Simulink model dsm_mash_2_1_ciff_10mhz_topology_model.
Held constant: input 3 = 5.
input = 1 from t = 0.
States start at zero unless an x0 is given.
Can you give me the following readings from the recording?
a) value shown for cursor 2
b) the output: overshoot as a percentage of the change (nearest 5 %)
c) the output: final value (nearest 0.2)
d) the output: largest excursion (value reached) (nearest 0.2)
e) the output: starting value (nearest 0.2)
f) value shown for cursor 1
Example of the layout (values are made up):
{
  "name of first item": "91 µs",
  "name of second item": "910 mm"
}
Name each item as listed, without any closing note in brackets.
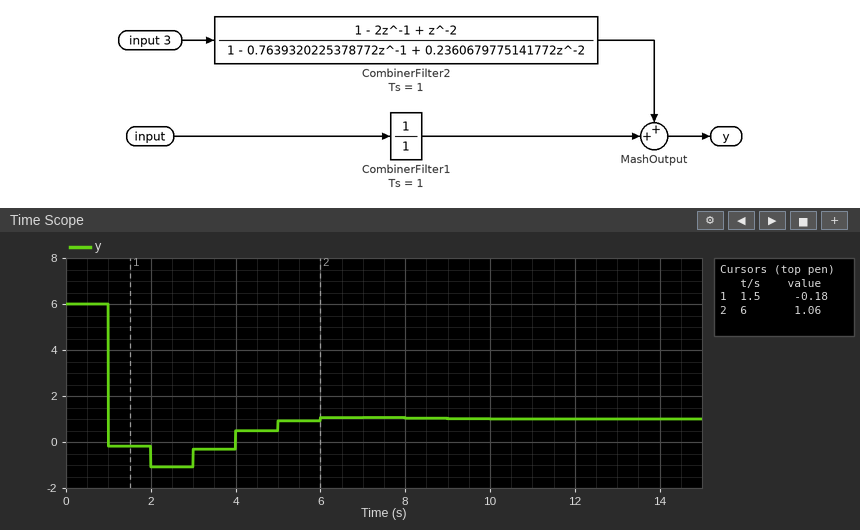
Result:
{
  "value shown for cursor 2": "1.06",
  "the output: overshoot as a percentage of the change": "40 %",
  "the output: final value": "1.0",
  "the output: largest excursion (value reached)": "-1.0",
  "the output: starting value": "6.0",
  "value shown for cursor 1": "-0.18"
}
